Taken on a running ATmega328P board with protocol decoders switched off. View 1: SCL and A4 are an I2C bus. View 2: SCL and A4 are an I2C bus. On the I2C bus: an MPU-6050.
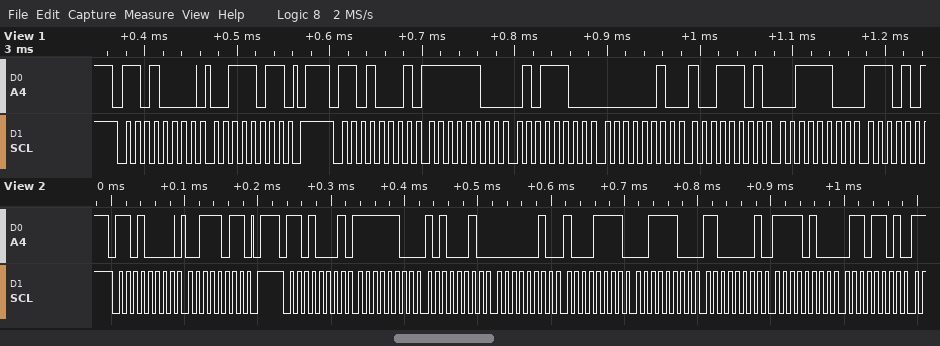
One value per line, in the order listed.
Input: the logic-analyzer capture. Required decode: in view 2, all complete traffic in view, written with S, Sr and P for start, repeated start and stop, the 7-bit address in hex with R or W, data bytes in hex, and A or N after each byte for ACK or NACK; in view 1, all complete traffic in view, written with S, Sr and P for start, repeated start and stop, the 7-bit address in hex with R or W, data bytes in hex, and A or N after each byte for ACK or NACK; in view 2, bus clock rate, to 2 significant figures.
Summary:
S 68W A 3B A P S 68R A FC A A2 A 02 A 8F A 3C A C1 A F4 A 6D A
S 68W A 3B A P S 68R A FC A 5C A 02 A 9D A 3C A
100 kHz
